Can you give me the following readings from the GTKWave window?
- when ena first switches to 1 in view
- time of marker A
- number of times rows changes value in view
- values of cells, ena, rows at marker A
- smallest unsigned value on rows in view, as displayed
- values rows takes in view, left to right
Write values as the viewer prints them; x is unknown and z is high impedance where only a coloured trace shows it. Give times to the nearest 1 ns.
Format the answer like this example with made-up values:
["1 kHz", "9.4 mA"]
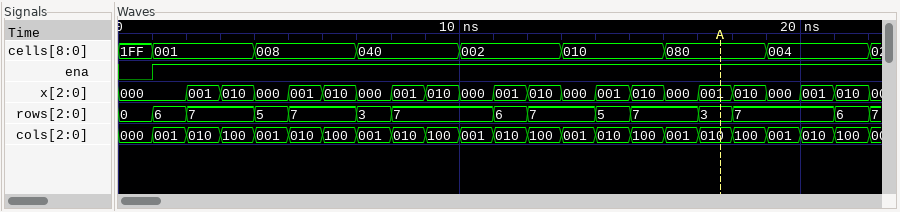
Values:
["1 ns", "18 ns", "14", "cells=080, ena=1, rows=3", "0", "0, 6, 7, 5, 7, 3, 7, 6, 7, 5, 7, 3, 7, 6, 7"]
